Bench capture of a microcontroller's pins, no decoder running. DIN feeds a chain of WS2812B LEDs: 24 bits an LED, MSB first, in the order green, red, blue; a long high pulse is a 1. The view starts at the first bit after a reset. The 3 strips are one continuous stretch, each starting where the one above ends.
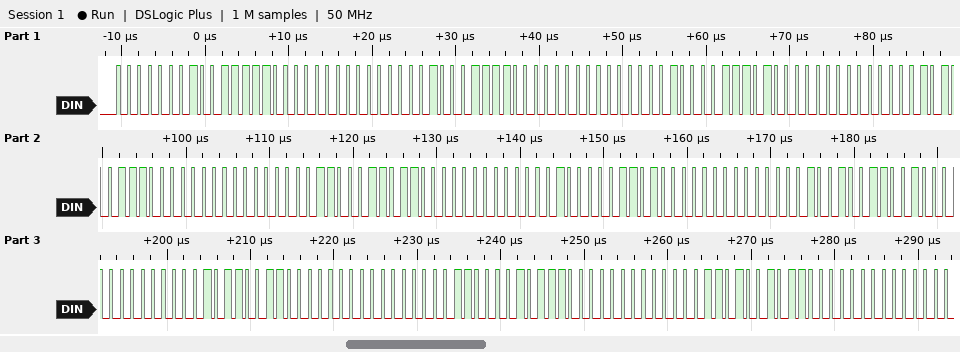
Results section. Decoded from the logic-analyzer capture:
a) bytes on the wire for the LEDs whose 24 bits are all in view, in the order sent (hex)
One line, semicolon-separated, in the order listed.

01 3E 00 02 3C 00 04 3A 00 05 38 00 06 36 00 08 34 00 09 32 00 0B 30 00 0C 2E 00 0D 2C 00
